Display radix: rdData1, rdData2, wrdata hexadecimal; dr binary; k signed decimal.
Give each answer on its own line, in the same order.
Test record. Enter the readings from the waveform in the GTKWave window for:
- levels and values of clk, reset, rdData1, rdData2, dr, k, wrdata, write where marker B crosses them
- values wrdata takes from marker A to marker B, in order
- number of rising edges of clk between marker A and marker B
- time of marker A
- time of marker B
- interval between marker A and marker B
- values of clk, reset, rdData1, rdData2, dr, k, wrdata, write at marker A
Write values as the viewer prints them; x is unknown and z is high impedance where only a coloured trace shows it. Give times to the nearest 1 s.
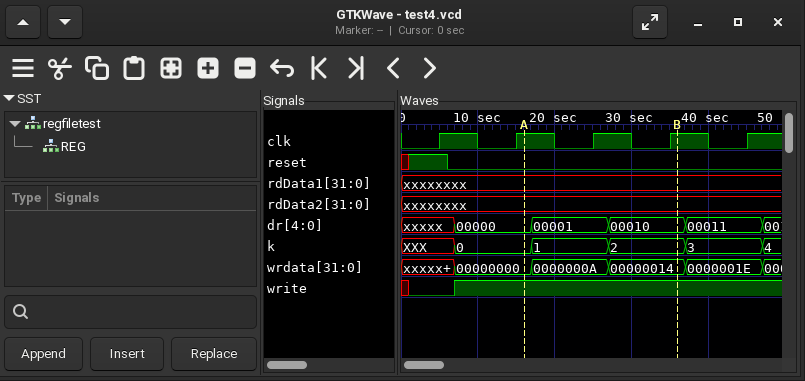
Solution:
clk=1, reset=0, rdData1=xxxxxxxx, rdData2=xxxxxxxx, dr=00010, k=2, wrdata=00000014, write=1
00000000, 0000000A, 00000014
2
16 s
36 s
20 s
clk=1, reset=0, rdData1=xxxxxxxx, rdData2=xxxxxxxx, dr=00000, k=0, wrdata=00000000, write=1
